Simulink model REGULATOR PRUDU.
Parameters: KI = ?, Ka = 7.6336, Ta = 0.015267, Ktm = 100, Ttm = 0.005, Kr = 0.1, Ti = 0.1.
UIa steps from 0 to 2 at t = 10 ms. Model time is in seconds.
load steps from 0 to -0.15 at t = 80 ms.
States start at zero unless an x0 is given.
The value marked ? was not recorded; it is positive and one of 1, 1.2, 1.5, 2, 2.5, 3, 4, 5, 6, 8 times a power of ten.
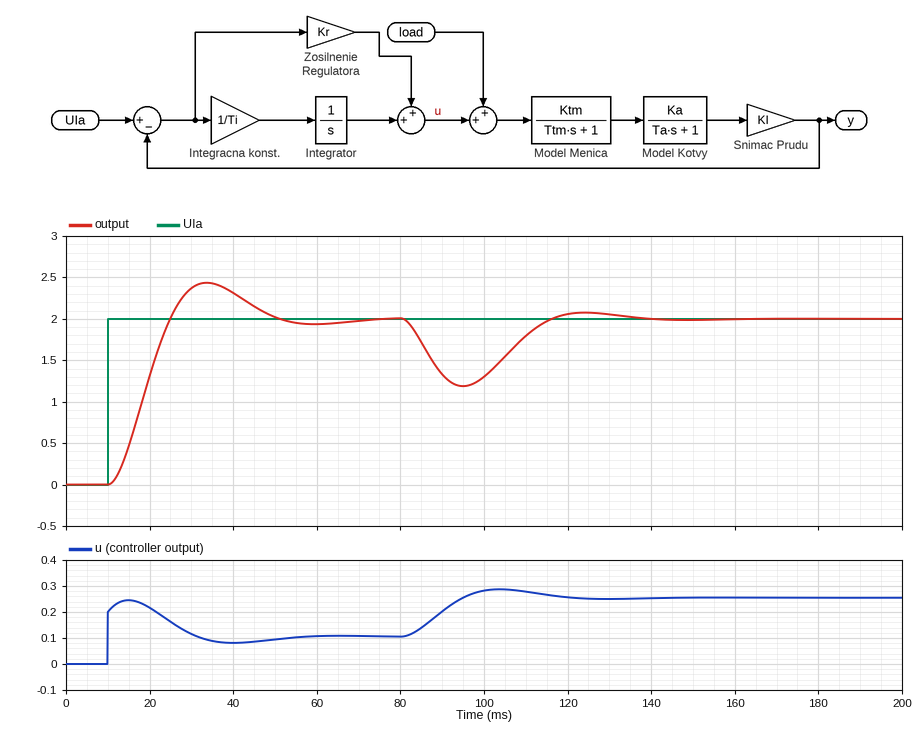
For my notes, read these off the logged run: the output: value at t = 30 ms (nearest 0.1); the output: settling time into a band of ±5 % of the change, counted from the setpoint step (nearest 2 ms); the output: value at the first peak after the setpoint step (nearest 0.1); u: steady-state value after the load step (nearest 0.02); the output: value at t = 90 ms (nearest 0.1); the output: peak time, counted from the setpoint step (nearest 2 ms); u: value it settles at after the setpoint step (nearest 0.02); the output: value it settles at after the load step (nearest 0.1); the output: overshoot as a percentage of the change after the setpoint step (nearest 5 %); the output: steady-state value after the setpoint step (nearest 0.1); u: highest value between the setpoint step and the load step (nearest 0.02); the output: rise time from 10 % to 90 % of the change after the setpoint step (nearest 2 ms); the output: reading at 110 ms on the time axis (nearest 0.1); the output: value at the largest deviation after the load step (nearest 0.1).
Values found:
2.4
36 ms
2.4
0.26
1.3
24 ms
0.10
2.0
20 %
2.0
0.24
10 ms
1.8
1.2
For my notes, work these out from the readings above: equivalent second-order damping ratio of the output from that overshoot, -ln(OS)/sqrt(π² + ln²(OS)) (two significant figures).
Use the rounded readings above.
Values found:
0.46
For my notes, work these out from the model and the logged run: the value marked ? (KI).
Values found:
0.025
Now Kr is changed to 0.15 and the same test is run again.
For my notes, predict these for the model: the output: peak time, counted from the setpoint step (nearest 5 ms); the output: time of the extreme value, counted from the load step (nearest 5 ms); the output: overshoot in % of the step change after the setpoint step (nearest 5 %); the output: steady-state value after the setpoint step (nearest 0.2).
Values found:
20 ms
15 ms
15 %
2.0
